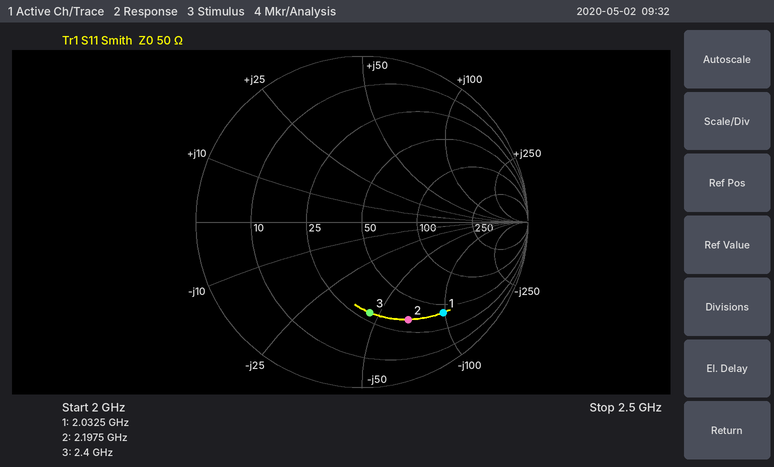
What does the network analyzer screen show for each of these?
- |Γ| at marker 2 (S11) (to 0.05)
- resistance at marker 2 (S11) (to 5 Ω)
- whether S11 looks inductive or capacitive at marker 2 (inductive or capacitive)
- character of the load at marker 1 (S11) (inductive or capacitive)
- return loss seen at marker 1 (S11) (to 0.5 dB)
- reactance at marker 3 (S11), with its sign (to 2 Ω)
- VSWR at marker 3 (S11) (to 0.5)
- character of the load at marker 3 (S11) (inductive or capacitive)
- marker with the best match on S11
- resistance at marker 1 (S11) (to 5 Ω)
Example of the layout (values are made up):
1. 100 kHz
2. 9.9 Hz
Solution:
1. 0.65
2. 35 Ω
3. capacitive
4. capacitive
5. 2.5 dB
6. -46 Ω
7. 3.5
8. capacitive
9. marker 3
10. 40 Ω
